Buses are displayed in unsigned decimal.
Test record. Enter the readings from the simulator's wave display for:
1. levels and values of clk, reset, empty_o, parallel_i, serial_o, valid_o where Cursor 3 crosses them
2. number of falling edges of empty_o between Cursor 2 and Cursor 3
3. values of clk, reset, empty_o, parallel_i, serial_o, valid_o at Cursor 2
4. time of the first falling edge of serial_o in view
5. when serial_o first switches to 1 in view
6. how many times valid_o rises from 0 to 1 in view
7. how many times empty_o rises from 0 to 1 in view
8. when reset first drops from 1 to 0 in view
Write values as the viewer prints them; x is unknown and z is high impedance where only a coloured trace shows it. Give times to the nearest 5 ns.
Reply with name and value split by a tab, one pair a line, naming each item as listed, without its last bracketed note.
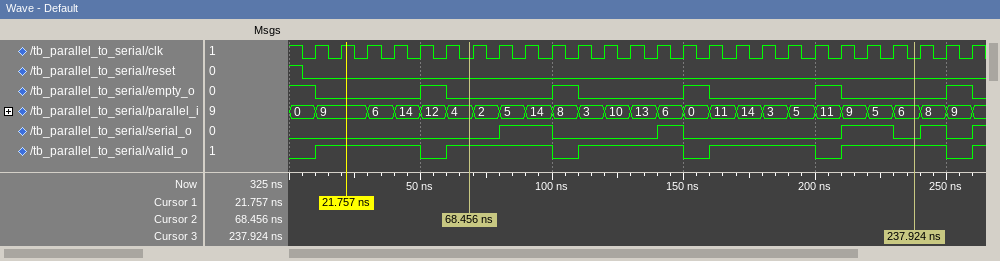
levels and values of clk, reset, empty_o, parallel_i, serial_o, valid_o where Cursor 3 crosses them	clk=0, reset=0, empty_o=0, parallel_i=6, serial_o=0, valid_o=1
number of falling edges of empty_o between Cursor 2 and Cursor 3	3
values of clk, reset, empty_o, parallel_i, serial_o, valid_o at Cursor 2	clk=0, reset=0, empty_o=0, parallel_i=4, serial_o=0, valid_o=1
time of the first falling edge of serial_o in view	100 ns
when serial_o first switches to 1 in view	80 ns
how many times valid_o rises from 0 to 1 in view	6
how many times empty_o rises from 0 to 1 in view	5
when reset first drops from 1 to 0 in view	5 ns
